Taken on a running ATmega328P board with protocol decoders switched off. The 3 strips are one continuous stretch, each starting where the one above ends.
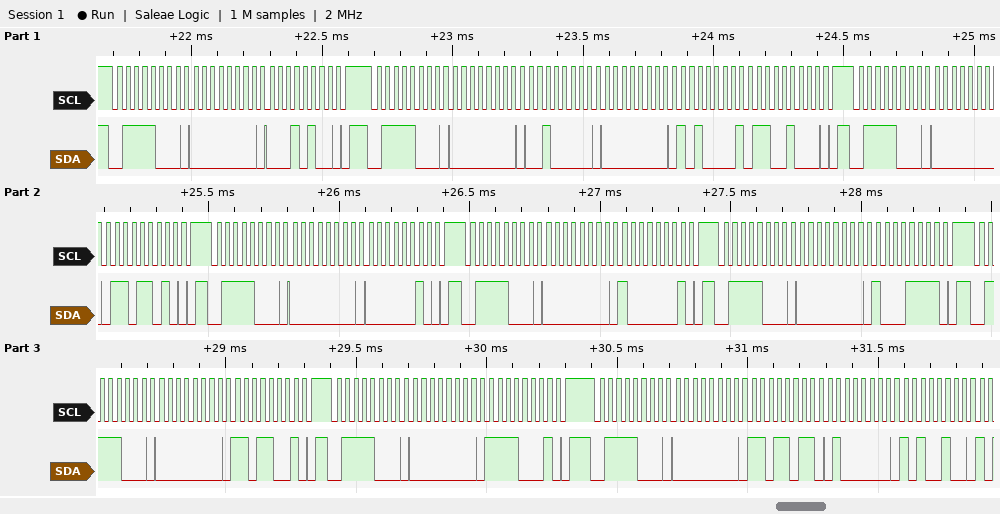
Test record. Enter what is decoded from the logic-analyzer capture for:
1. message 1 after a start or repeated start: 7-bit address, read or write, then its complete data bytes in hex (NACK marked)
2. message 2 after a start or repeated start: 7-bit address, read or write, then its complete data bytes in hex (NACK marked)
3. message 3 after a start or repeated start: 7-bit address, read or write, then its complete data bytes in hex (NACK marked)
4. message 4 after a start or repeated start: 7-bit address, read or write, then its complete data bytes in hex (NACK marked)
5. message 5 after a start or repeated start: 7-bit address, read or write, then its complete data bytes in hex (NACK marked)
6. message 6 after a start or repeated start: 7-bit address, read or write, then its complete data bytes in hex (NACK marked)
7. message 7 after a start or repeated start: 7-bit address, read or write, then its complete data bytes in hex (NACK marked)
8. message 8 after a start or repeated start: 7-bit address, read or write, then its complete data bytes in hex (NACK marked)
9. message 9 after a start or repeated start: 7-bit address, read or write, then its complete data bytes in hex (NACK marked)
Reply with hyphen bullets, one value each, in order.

- 0x3C write: 00 14
- 0x3C write: 00 20 00 A1 C8
- 0x3C write: 00 DA
- 0x3C write: 00 02
- 0x3C write: 00 81
- 0x3C write: 00 8F
- 0x3C write: 00 D9
- 0x3C write: 00 F1
- 0x3C write: 00 DB 40 A4
